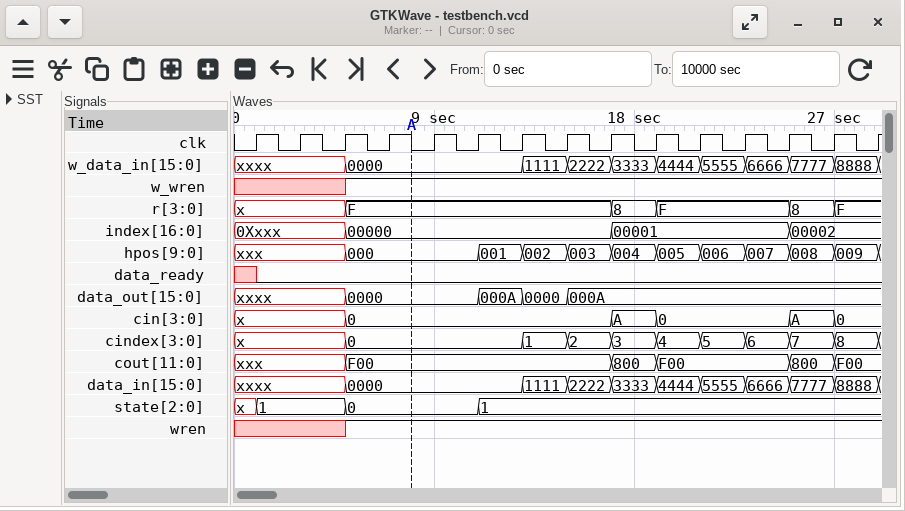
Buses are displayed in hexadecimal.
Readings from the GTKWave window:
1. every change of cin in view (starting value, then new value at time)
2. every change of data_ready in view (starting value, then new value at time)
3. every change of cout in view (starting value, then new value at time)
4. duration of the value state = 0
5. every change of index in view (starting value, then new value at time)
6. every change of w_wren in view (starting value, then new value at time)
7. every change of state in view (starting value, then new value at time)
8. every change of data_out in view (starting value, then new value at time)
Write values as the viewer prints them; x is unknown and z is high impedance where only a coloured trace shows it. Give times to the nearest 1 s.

x, 0 at 5 s, A at 17 s, 0 at 19 s, A at 25 s, 0 at 27 s
x, 0 at 1 s
xxx, F00 at 5 s, 800 at 17 s, F00 at 19 s, 800 at 25 s, F00 at 27 s
6 s
0Xxxx, 00000 at 5 s, 00001 at 17 s, 00002 at 25 s
x, 1 at 5 s
x, 1 at 1 s, 0 at 5 s, 1 at 11 s
xxxx, 0000 at 5 s, 000A at 11 s, 0000 at 13 s, 000A at 15 s
